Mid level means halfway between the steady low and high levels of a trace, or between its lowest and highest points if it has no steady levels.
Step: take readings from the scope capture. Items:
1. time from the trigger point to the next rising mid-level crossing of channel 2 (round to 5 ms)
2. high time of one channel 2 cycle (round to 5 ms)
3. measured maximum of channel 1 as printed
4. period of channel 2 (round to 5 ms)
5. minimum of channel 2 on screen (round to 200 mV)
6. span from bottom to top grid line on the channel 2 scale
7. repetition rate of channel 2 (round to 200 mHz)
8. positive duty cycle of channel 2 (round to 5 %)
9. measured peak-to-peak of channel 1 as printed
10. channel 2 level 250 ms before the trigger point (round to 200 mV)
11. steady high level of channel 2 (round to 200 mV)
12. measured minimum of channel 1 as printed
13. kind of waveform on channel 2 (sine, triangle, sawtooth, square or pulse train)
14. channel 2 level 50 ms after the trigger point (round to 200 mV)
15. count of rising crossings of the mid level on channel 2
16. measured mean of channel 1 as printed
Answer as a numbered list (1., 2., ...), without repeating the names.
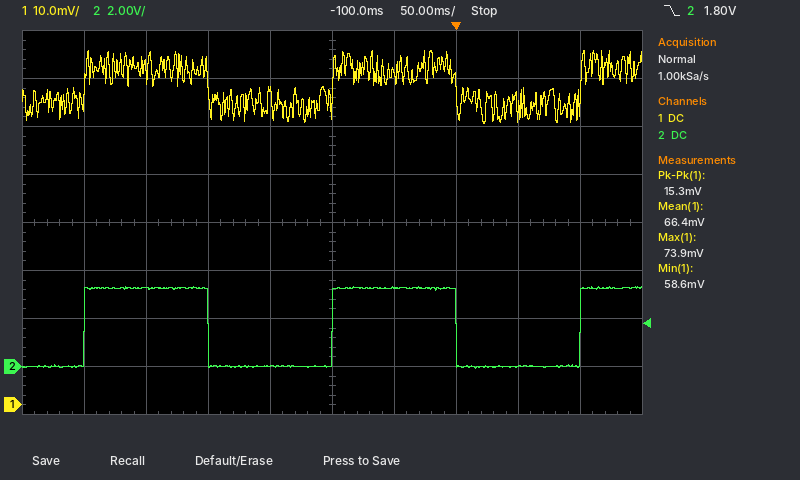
1. 100 ms
2. 100 ms
3. 73.9 mV
4. 200 ms
5. 0.0 V
6. 16 V
7. 5.0 Hz
8. 50 %
9. 15.3 mV
10. 3.2 V
11. 3.2 V
12. 58.6 mV
13. square
14. 0.0 V
15. 3
16. 66.4 mV
